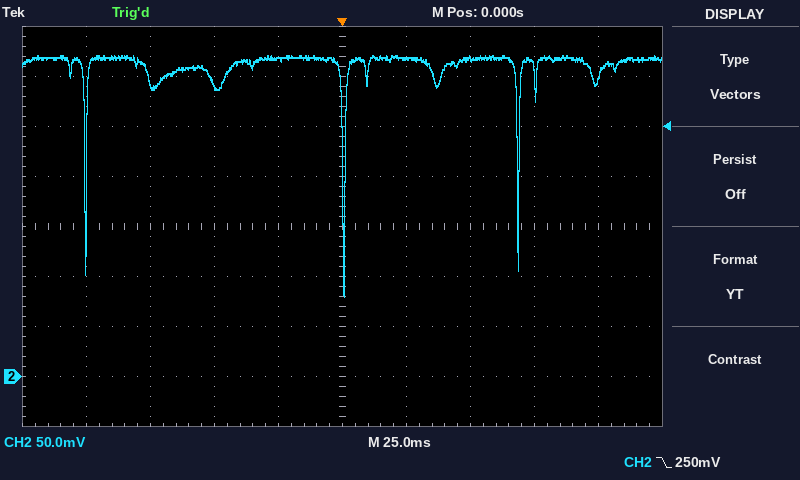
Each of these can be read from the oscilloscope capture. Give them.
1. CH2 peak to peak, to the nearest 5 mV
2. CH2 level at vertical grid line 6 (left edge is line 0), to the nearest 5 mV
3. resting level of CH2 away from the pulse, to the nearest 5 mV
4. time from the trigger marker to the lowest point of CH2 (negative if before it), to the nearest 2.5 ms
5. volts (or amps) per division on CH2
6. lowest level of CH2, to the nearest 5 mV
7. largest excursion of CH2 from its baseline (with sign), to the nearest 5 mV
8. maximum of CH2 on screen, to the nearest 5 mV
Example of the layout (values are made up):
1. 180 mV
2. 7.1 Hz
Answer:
1. 240 mV
2. 320 mV
3. 320 mV
4. 0.0 ms
5. 50 mV
6. 80 mV
7. -240 mV
8. 320 mV
